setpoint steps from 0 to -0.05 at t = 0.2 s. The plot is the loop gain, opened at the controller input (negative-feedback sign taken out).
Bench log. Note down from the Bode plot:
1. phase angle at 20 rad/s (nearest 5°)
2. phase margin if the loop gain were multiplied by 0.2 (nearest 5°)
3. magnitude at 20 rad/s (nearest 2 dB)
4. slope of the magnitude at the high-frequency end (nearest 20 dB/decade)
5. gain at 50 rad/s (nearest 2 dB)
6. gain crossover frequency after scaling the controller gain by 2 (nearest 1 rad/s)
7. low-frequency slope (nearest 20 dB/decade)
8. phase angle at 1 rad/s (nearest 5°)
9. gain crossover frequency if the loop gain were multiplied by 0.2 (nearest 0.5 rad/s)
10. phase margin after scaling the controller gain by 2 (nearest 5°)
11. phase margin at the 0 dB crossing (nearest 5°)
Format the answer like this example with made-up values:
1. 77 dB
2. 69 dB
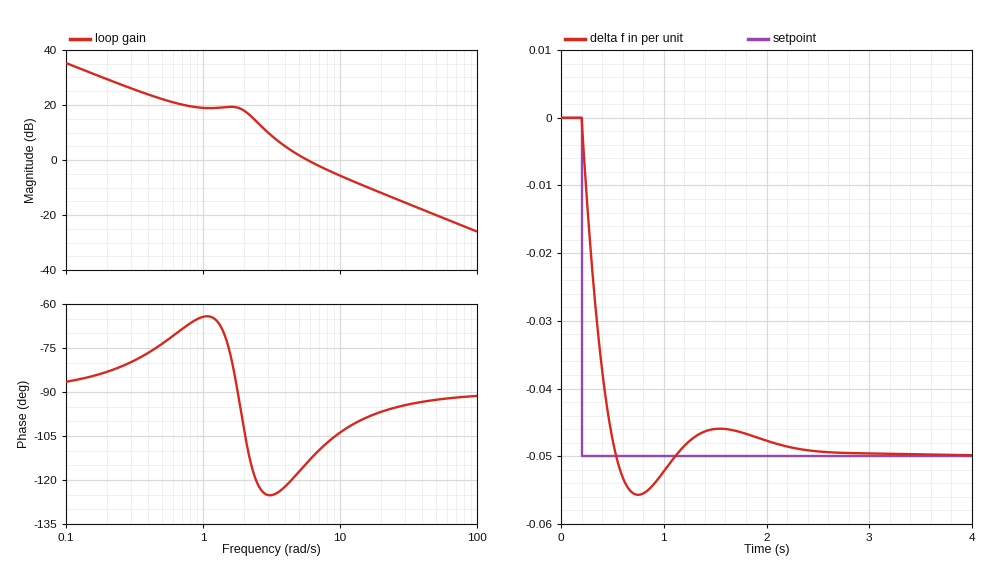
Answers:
1. -95°
2. 60°
3. -12 dB
4. -20 dB/decade
5. -20 dB
6. 10 rad/s
7. -20 dB/decade
8. -65°
9. 2.5 rad/s
10. 75°
11. 65°
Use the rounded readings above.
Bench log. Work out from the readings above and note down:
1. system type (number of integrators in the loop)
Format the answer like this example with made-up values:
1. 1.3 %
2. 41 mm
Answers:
1. 1
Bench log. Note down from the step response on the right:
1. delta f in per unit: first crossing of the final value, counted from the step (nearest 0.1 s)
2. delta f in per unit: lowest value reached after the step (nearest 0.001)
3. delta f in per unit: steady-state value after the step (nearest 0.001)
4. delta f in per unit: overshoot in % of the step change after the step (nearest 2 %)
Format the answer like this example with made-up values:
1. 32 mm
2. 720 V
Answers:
1. 0.3 s
2. -0.056
3. -0.050
4. 12 %
